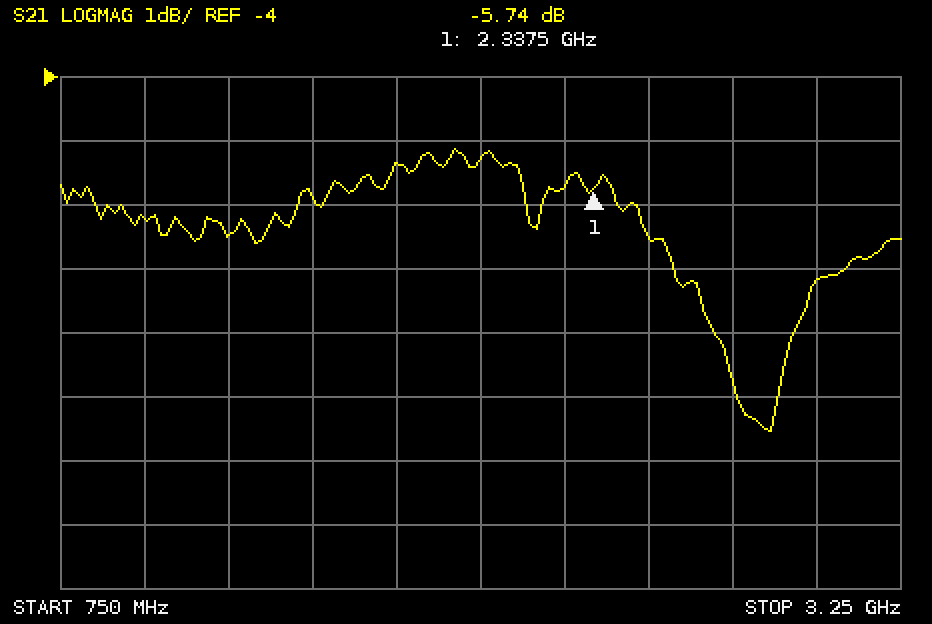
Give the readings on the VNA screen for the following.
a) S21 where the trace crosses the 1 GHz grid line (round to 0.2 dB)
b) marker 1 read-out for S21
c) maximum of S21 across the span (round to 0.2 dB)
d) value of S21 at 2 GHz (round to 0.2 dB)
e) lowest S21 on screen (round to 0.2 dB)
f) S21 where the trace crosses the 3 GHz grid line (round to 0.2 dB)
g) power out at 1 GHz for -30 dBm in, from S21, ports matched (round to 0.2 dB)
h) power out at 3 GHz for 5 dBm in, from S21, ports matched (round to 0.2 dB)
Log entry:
-6.2 dB
-5.74 dB
-5.2 dB
-5.2 dB
-9.6 dB
-7.2 dB
-36.2 dBm
-2.2 dBm
